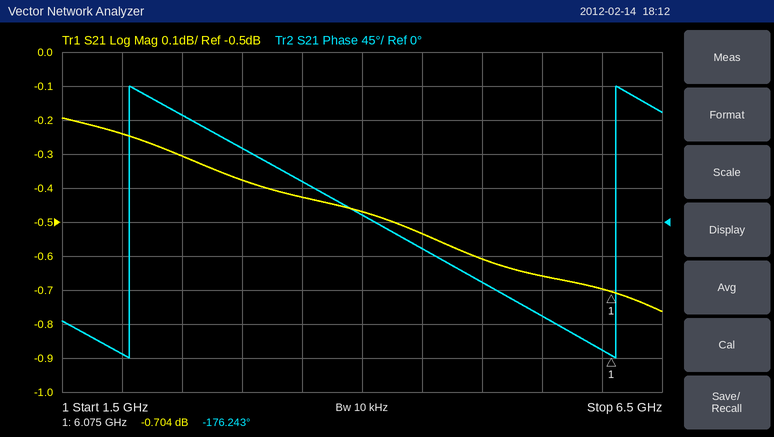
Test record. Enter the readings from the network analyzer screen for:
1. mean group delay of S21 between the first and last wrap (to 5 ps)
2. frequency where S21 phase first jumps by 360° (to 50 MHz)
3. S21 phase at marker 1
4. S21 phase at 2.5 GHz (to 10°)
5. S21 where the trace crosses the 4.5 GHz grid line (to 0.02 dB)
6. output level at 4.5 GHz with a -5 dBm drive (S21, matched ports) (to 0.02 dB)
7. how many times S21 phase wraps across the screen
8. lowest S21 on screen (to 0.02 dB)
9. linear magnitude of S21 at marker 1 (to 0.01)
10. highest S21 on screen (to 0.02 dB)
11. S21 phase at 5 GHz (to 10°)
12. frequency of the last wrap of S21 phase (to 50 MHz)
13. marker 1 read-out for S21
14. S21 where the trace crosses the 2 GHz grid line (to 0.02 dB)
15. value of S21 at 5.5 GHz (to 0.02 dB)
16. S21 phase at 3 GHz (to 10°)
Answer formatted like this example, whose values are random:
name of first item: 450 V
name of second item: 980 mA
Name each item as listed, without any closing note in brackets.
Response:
mean group delay of S21 between the first and last wrap: 245 ps
frequency where S21 phase first jumps by 360°: 2.05 GHz
S21 phase at marker 1: -176.243°
S21 phase at 2.5 GHz: 140°
S21 where the trace crosses the 4.5 GHz grid line: -0.54 dB
output level at 4.5 GHz with a -5 dBm drive (S21, matched ports): -5.54 dBm
how many times S21 phase wraps across the screen: 2
lowest S21 on screen: -0.76 dB
linear magnitude of S21 at marker 1: 0.92
highest S21 on screen: -0.20 dB
S21 phase at 5 GHz: -80°
frequency of the last wrap of S21 phase: 6.10 GHz
marker 1 read-out for S21: -0.704 dB
S21 where the trace crosses the 2 GHz grid line: -0.24 dB
value of S21 at 5.5 GHz: -0.66 dB
S21 phase at 3 GHz: 100°
